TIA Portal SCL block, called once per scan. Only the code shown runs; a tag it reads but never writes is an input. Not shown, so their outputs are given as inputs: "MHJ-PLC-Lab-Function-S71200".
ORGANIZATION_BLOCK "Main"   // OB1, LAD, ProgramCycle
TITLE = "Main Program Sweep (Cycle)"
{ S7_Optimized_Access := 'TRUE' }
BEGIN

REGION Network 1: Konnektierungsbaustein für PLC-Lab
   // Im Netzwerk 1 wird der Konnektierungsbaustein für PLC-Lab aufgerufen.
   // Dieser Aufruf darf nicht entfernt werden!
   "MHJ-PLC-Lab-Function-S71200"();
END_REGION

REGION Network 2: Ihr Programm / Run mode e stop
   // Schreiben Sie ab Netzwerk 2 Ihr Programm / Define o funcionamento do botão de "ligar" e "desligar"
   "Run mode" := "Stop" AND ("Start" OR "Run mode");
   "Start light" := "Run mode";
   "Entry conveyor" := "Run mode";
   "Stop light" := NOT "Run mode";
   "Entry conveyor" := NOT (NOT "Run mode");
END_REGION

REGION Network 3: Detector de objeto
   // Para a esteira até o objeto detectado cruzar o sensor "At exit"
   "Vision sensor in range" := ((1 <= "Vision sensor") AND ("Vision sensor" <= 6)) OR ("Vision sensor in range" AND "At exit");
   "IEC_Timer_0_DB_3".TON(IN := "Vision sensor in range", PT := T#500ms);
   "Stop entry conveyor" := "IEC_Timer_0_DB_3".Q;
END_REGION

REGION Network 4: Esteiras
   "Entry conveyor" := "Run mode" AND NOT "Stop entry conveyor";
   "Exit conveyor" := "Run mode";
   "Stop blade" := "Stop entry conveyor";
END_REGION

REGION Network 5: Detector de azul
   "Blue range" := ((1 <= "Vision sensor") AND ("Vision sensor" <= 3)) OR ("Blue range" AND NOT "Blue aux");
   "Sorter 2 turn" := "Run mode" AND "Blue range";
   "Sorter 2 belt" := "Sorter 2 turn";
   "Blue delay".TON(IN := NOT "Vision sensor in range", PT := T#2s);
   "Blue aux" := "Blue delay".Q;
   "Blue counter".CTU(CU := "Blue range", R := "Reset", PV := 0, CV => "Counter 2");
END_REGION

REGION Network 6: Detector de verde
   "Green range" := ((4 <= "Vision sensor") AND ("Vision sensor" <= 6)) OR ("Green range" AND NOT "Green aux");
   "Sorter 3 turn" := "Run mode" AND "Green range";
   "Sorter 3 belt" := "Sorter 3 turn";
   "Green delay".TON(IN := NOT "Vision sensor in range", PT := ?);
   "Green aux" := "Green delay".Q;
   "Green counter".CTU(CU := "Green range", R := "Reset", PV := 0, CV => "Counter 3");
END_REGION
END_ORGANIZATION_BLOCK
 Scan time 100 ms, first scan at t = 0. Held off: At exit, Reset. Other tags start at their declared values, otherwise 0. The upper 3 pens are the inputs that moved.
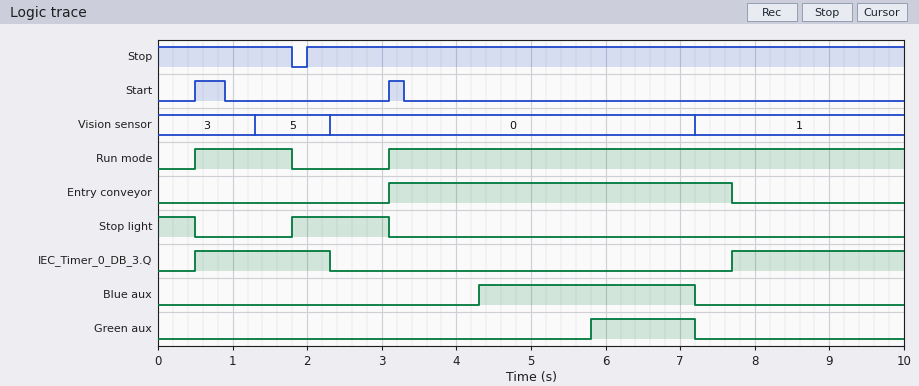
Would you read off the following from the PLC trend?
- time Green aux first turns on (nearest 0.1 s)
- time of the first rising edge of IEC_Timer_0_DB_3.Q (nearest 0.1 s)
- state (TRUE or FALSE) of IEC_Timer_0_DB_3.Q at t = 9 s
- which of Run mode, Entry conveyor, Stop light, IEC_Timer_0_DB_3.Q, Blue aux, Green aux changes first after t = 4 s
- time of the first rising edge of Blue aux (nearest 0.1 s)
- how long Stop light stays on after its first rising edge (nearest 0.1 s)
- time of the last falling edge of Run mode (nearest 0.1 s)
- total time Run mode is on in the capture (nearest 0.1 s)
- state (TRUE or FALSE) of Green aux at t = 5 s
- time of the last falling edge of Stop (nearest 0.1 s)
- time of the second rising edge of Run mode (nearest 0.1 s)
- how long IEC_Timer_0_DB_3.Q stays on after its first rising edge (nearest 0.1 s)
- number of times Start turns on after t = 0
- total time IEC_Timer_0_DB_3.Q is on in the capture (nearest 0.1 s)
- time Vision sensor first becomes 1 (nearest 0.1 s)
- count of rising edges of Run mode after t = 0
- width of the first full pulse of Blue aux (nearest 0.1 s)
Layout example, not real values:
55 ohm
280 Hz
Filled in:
5.8 s
0.5 s
TRUE
Blue aux
4.3 s
1.3 s
1.8 s
8.2 s
FALSE
1.8 s
3.1 s
1.8 s
2
4.1 s
7.2 s
2
2.9 s
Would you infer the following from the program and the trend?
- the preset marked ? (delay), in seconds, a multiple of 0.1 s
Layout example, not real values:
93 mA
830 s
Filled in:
3.5 s
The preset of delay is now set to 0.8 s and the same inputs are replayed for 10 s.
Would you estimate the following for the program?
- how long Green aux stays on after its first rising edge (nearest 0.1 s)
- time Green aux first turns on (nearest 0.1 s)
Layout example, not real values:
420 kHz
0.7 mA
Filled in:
4.1 s
3.1 s
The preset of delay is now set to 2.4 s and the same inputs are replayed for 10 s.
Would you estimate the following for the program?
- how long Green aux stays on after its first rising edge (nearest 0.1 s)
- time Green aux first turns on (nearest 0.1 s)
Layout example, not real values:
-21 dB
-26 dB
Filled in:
2.5 s
4.7 s
